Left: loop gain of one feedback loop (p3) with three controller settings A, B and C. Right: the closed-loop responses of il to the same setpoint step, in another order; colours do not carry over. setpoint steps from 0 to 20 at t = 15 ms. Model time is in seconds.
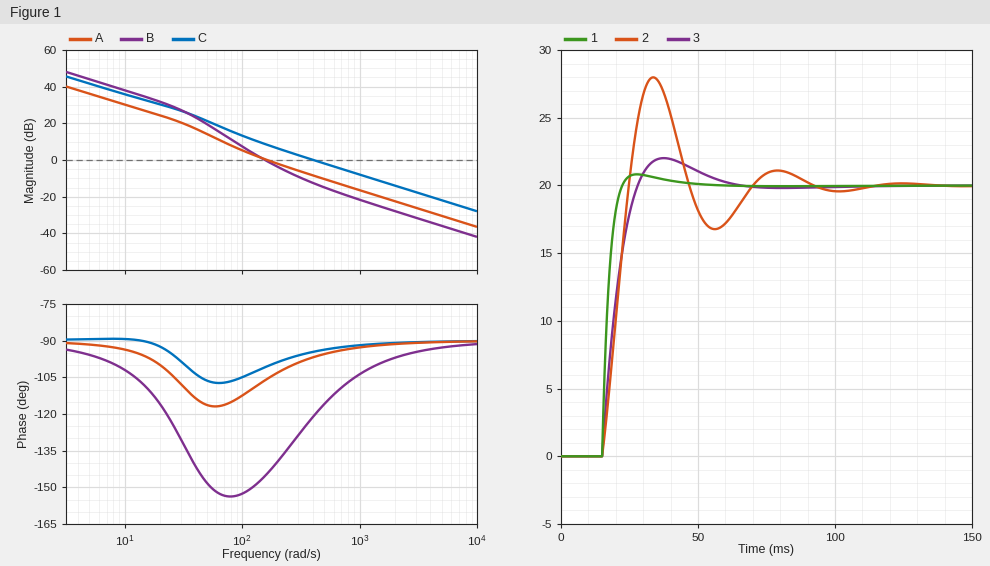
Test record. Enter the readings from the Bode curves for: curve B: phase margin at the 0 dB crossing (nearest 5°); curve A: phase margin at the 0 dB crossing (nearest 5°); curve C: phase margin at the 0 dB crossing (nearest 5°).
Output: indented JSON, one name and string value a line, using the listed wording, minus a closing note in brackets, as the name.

{
  "curve B: phase margin at the 0 dB crossing": "35°",
  "curve A: phase margin at the 0 dB crossing": "75°",
  "curve C: phase margin at the 0 dB crossing": "85°"
}
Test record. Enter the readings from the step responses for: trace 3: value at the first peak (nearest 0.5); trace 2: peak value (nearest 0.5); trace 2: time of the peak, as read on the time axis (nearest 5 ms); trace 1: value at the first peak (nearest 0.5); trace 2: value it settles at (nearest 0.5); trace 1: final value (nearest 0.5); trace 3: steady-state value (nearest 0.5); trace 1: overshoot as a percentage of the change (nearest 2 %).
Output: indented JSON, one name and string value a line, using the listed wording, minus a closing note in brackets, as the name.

{
  "trace 3: value at the first peak": "22.0",
  "trace 2: peak value": "28.0",
  "trace 2: time of the peak, as read on the time axis": "35 ms",
  "trace 1: value at the first peak": "21.0",
  "trace 2: value it settles at": "20.0",
  "trace 1: final value": "20.0",
  "trace 3: steady-state value": "20.0",
  "trace 1: overshoot as a percentage of the change": "4 %"
}
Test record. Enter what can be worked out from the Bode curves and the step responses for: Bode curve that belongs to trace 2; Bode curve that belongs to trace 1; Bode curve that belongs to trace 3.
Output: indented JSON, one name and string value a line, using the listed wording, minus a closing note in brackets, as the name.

{
  "Bode curve that belongs to trace 2": "B",
  "Bode curve that belongs to trace 1": "C",
  "Bode curve that belongs to trace 3": "A"
}
